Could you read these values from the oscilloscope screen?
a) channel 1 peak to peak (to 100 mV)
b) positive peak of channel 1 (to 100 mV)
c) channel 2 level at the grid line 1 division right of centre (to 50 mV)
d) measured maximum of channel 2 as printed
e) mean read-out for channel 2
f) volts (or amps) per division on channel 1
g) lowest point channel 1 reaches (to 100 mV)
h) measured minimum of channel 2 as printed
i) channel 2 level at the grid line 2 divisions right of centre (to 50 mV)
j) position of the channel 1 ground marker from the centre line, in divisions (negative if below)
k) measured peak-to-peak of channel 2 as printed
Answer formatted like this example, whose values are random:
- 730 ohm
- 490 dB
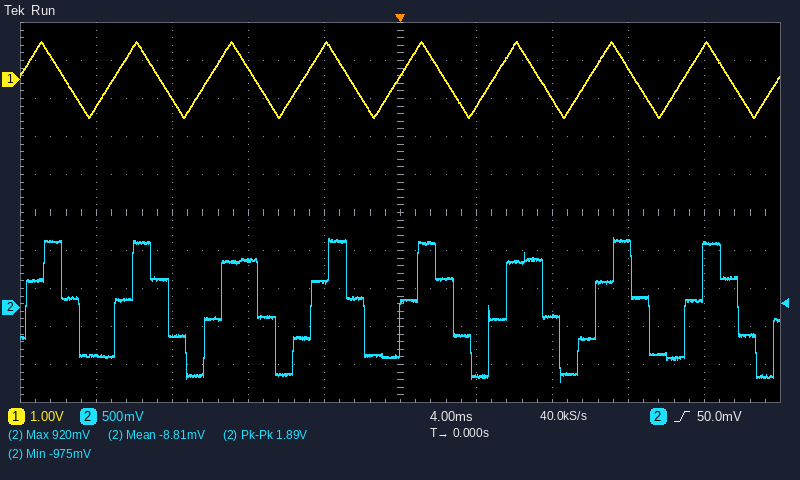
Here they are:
- 2.0 V
- 1.0 V
- -900 mV
- 920 mV
- -8.81 mV
- 1 V
- -1.0 V
- -975 mV
- -100 mV
- +3.5 div
- 1.89 V
